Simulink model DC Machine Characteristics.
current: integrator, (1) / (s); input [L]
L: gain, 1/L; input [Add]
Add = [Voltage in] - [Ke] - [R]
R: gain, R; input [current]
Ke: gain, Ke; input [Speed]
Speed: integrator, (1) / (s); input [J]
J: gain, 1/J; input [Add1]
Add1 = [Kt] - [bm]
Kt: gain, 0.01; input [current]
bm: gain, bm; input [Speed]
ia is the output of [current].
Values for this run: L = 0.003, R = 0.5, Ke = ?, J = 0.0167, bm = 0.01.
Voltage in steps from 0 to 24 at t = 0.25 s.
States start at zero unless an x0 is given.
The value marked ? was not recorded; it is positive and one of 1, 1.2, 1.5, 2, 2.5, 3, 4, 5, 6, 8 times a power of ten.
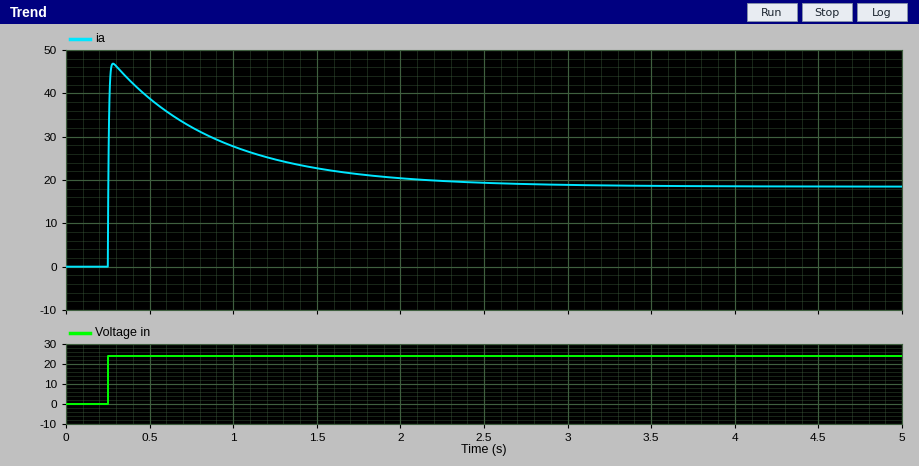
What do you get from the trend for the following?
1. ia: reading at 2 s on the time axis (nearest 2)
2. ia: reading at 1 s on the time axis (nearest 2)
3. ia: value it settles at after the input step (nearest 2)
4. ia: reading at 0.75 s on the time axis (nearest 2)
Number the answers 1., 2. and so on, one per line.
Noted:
1. 20
2. 28
3. 18
4. 32
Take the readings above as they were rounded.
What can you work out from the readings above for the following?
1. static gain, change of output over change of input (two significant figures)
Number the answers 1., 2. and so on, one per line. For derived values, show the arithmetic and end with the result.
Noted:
1. (18 - 0) / (24 - 0) = 0.75
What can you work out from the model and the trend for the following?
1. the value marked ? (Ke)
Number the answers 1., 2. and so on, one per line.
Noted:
1. 0.8
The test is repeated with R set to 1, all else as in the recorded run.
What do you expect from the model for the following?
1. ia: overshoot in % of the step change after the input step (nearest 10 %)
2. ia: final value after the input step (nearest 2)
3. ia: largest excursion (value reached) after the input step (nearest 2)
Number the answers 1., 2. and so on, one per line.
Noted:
1. 80 %
2. 14
3. 24
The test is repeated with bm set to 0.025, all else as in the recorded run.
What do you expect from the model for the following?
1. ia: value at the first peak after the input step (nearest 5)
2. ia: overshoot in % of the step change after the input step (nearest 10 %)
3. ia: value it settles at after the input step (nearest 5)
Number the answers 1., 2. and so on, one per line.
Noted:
1. 45
2. 60 %
3. 30
